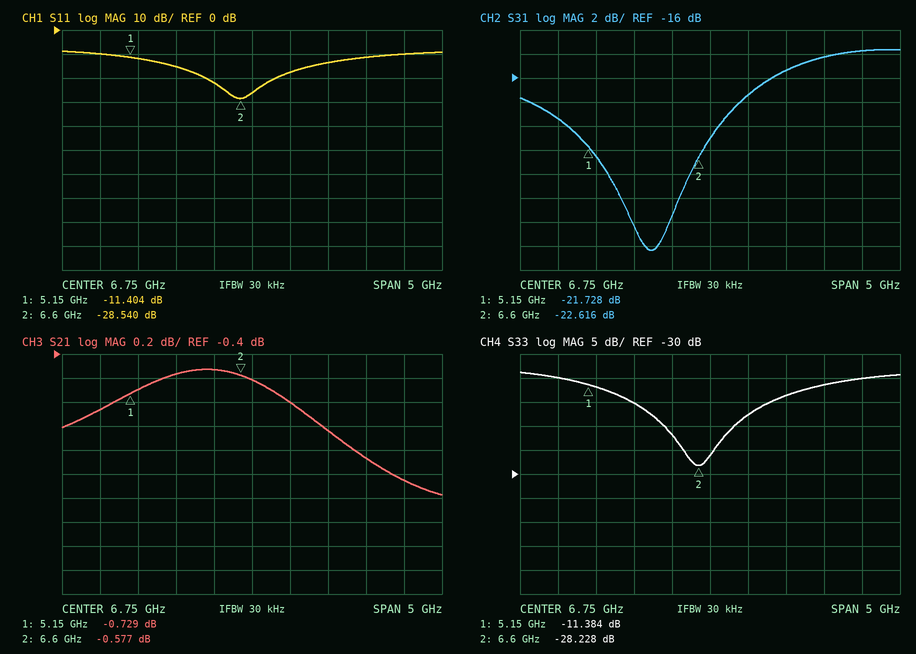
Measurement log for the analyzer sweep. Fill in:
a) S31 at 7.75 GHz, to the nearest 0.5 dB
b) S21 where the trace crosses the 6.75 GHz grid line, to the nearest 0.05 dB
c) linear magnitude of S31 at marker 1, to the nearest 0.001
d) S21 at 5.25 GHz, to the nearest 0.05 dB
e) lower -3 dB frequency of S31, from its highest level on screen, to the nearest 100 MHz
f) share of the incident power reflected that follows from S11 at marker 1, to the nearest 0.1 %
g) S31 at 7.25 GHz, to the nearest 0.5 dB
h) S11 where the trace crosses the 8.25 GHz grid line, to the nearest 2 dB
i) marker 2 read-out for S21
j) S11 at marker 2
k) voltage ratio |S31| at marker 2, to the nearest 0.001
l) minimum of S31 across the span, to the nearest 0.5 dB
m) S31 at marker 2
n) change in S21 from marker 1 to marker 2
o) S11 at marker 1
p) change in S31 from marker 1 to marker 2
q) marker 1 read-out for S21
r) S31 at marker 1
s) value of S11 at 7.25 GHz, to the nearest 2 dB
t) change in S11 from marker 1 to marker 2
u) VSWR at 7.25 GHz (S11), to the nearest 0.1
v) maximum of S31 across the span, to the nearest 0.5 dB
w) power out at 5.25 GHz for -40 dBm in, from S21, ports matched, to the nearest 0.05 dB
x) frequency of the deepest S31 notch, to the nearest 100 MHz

-15.5 dB
-0.60 dB
0.082
-0.70 dB
7.4 GHz
7.2 %
-17.5 dB
-12 dB
-0.577 dB
-28.540 dB
0.074
-30.5 dB
-22.616 dB
0.152 dB
-11.404 dB
-0.888 dB
-0.729 dB
-21.728 dB
-18 dB
-17.136 dB
1.3
-13.5 dB
-40.70 dBm
6.0 GHz
